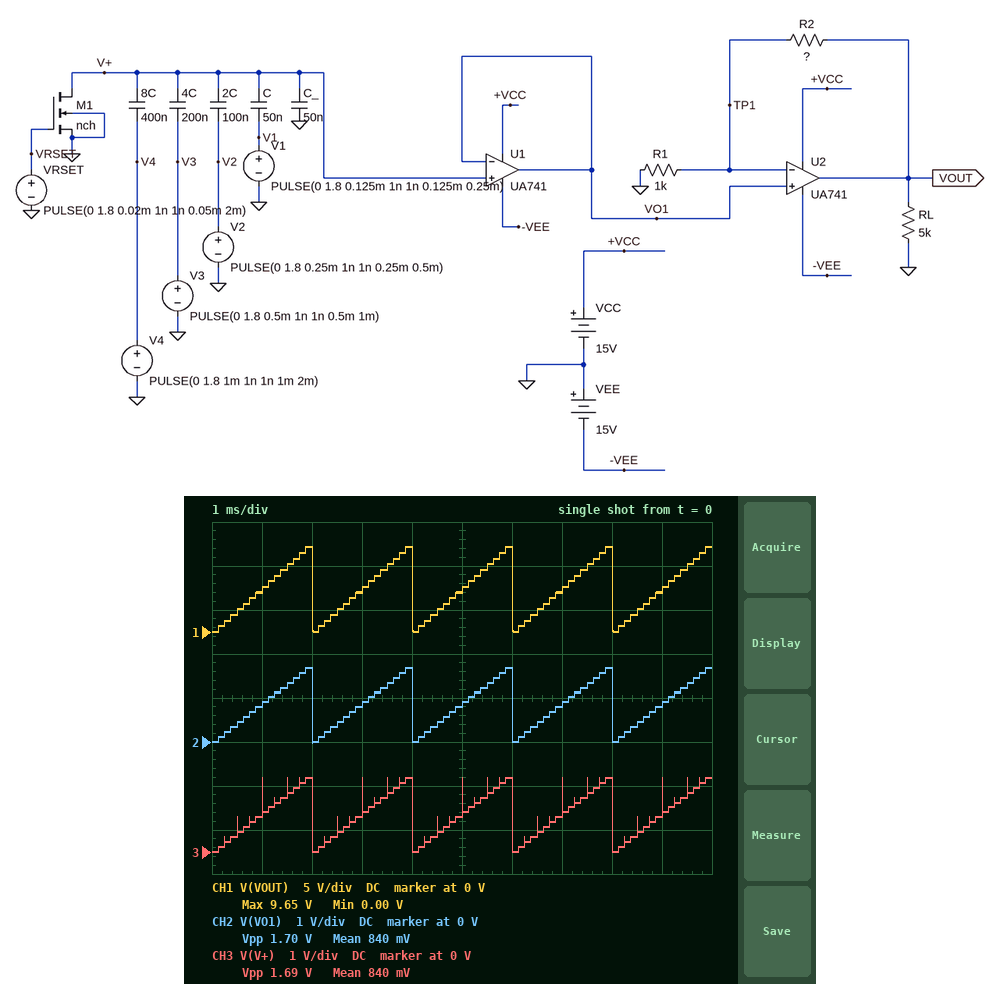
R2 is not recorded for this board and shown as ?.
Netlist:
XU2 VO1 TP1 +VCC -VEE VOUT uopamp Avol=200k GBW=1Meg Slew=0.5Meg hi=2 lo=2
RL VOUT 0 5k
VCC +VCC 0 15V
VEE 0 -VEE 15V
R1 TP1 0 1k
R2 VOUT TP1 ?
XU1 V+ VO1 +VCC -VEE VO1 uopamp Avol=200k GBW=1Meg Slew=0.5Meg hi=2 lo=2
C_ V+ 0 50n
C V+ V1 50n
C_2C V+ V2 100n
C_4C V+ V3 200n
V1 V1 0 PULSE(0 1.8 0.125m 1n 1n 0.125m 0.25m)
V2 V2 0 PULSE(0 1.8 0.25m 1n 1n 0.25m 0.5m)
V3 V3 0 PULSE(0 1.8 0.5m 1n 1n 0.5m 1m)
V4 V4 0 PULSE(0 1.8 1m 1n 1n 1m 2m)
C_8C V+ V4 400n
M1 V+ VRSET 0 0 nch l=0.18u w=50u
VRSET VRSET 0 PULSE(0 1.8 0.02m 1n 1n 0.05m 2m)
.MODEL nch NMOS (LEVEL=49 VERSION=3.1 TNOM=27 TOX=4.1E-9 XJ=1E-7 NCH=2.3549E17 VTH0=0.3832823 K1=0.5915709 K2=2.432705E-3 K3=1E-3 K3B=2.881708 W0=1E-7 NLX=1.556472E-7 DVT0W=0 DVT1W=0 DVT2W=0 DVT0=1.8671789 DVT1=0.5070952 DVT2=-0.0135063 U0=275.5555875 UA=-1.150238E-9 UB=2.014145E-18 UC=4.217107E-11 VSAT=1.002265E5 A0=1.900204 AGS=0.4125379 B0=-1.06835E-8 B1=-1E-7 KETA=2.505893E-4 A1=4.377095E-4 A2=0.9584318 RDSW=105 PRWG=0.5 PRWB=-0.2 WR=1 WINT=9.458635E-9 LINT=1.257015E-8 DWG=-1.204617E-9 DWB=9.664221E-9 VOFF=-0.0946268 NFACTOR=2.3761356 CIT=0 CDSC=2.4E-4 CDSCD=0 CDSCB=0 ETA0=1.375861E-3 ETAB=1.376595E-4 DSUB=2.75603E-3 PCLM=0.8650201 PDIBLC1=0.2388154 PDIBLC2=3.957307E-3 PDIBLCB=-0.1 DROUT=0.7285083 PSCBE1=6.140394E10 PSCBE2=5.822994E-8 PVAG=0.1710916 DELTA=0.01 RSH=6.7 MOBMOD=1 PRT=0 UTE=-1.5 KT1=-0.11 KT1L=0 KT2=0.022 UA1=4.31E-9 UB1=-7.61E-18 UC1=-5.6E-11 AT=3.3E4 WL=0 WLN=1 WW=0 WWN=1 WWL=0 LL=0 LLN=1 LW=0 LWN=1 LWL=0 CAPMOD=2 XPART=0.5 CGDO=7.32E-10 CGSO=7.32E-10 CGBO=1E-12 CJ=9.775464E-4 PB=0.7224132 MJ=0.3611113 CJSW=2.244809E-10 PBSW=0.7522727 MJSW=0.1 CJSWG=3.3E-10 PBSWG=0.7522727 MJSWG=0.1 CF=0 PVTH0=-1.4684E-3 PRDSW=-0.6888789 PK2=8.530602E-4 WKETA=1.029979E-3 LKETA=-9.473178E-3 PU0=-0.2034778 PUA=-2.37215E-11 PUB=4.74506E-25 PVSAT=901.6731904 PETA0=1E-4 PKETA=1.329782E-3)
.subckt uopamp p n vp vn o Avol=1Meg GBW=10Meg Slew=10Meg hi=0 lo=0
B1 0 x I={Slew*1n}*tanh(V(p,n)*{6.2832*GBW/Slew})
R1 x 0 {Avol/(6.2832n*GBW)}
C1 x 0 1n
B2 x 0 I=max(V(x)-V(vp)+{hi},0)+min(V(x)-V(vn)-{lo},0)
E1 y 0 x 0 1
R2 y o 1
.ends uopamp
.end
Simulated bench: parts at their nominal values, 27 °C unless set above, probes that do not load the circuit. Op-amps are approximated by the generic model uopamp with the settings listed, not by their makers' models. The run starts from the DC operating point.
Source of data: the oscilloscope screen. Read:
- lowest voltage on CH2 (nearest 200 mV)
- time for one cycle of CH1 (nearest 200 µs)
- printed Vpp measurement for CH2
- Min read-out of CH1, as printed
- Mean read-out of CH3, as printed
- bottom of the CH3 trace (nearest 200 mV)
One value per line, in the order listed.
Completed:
0 V
2.0 ms
1.70 V
0.00 V
840 mV
0 V
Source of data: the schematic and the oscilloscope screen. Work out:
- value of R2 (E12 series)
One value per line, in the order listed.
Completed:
4.7 kΩ
